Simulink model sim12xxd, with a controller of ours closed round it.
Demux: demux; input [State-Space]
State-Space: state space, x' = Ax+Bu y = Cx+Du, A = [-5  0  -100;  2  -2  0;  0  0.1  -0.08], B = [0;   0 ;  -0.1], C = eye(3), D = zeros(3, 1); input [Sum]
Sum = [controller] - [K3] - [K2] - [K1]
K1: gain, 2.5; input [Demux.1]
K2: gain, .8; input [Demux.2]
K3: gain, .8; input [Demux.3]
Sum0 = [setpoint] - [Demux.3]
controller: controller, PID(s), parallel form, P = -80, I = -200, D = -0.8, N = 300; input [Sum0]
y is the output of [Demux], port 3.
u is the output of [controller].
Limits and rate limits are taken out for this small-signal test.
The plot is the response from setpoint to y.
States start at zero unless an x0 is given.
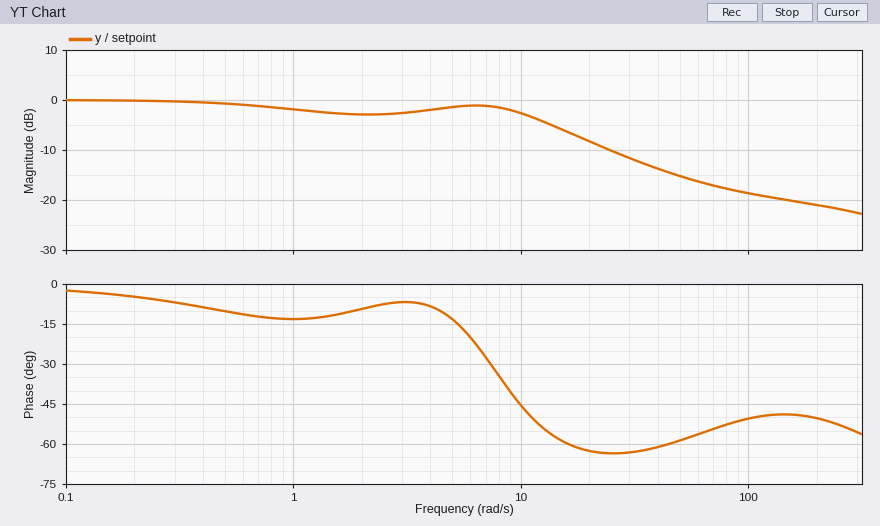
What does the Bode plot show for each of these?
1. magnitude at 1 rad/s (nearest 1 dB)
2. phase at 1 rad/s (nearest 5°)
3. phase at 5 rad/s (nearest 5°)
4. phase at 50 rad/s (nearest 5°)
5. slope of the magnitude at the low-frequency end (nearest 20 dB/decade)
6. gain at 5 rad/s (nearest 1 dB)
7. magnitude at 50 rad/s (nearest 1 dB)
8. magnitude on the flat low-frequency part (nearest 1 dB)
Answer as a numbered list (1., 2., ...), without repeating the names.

1. -2 dB
2. -15°
3. -15°
4. -60°
5. 0 dB/decade
6. -1 dB
7. -15 dB
8. 0 dB
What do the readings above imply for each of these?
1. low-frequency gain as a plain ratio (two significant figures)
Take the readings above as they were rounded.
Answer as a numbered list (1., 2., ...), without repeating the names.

1. 1.0
